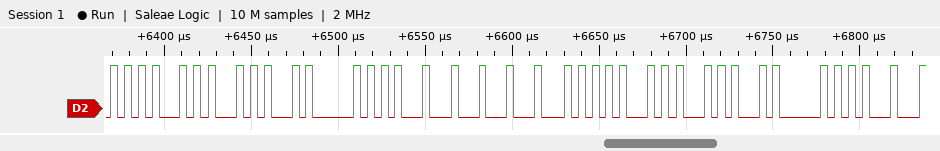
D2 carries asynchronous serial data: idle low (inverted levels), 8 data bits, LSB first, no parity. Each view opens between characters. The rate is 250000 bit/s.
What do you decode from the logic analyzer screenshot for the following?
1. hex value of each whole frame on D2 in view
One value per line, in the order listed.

D5, 75, 5D, D5, 77, 77, D5, 75, 5D, D5
